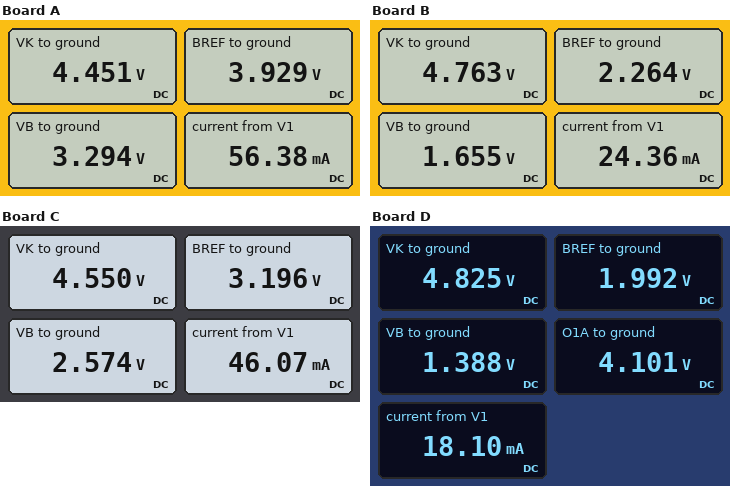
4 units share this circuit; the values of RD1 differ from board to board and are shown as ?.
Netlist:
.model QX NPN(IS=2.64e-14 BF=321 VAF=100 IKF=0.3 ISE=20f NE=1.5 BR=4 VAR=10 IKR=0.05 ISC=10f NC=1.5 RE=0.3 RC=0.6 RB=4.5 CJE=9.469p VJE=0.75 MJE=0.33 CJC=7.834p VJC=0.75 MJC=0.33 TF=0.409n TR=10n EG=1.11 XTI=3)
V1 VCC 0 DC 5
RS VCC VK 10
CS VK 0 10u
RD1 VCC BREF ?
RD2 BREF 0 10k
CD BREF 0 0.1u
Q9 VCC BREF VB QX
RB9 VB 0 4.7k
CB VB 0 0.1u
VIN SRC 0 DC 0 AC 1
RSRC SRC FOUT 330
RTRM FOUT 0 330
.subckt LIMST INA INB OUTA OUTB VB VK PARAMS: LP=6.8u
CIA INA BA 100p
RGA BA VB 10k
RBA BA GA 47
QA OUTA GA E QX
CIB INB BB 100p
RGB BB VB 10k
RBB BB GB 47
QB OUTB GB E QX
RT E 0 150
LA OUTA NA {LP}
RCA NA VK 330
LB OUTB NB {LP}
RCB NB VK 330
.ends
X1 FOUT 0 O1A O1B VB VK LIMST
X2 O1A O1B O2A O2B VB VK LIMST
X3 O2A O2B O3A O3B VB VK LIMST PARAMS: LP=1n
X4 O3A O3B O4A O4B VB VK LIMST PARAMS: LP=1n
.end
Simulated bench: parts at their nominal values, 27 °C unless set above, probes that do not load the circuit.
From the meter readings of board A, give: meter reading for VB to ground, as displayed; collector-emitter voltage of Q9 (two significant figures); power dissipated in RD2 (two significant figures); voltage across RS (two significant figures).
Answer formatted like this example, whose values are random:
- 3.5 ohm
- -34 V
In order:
- 3.294 V
- 1.7 V
- 1.5 mW
- 550 mV
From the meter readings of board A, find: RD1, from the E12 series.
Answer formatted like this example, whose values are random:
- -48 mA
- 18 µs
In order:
- 2.7 kΩ
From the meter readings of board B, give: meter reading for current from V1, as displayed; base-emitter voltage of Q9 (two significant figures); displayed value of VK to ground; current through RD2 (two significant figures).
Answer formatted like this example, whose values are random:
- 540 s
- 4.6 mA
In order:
- 24.36 mA
- 610 mV
- 4.763 V
- 230 µA
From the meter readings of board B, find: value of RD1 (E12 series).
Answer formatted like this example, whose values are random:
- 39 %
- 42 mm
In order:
- 12 kΩ
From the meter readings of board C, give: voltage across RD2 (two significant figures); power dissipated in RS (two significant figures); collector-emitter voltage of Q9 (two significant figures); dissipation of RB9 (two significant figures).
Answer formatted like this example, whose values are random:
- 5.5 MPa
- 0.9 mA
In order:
- 3.2 V
- 20 mW
- 2.4 V
- 1.4 mW
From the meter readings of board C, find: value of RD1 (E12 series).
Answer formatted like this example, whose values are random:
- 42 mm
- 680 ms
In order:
- 5.6 kΩ
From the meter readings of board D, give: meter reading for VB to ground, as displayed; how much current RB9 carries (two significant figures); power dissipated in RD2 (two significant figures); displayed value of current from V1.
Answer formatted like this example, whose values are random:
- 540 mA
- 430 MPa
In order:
- 1.388 V
- 300 µA
- 400 µW
- 18.10 mA
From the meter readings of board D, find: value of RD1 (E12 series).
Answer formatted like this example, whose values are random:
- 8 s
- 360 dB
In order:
- 15 kΩ
